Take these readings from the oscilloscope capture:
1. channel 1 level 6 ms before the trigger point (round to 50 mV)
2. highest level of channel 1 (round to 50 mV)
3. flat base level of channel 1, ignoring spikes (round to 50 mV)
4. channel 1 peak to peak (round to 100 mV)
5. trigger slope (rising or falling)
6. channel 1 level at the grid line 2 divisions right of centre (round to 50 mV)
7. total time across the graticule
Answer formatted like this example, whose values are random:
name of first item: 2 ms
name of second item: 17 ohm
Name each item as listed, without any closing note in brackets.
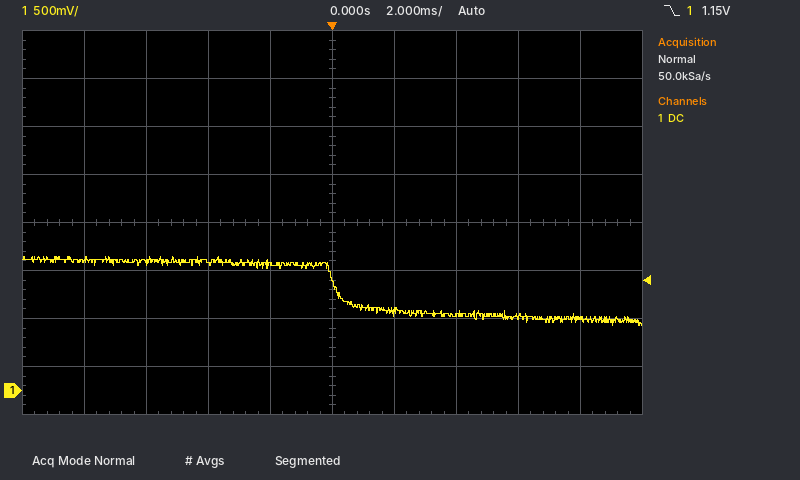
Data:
channel 1 level 6 ms before the trigger point: 1.35 V
highest level of channel 1: 1.40 V
flat base level of channel 1, ignoring spikes: 750 mV
channel 1 peak to peak: 700 mV
trigger slope: falling
channel 1 level at the grid line 2 divisions right of centre: 800 mV
total time across the graticule: 20 ms
